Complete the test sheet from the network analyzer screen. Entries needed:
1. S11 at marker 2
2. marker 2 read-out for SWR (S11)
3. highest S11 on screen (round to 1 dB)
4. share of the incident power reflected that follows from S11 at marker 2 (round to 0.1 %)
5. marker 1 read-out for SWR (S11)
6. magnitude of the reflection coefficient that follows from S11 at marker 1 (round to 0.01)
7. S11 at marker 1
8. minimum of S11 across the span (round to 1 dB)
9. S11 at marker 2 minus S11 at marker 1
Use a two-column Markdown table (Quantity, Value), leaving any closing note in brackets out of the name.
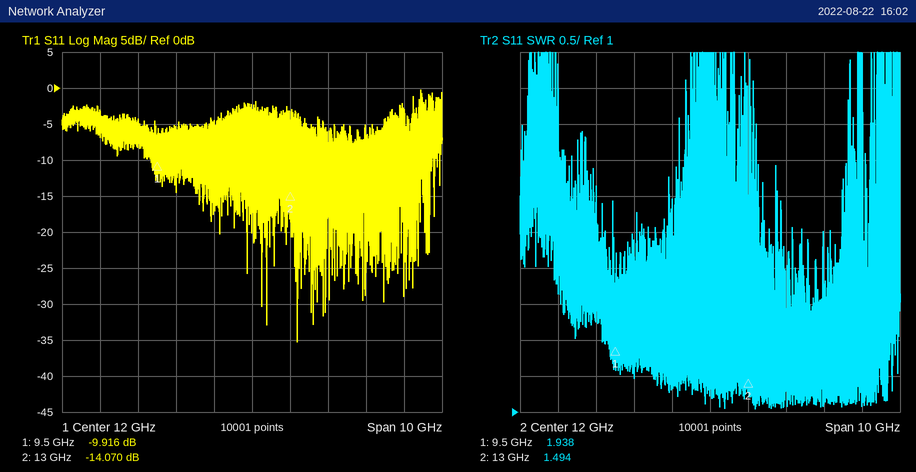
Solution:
| Quantity | Value |
|---|---|
| S11 at marker 2 | -14.070 dB |
| marker 2 read-out for SWR | 1.494 |
| highest S11 on screen | 0 dB |
| share of the incident power reflected that follows from S11 at marker 2 | 3.9 % |
| marker 1 read-out for SWR | 1.938 |
| magnitude of the reflection coefficient that follows from S11 at marker 1 | 0.32 |
| S11 at marker 1 | -9.916 dB |
| minimum of S11 across the span | -35 dB |
| S11 at marker 2 minus S11 at marker 1 | -4.154 dB |
